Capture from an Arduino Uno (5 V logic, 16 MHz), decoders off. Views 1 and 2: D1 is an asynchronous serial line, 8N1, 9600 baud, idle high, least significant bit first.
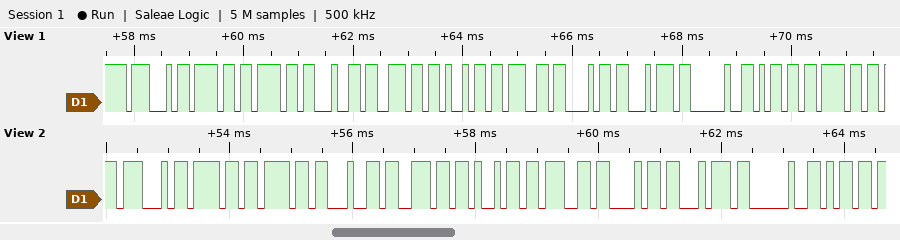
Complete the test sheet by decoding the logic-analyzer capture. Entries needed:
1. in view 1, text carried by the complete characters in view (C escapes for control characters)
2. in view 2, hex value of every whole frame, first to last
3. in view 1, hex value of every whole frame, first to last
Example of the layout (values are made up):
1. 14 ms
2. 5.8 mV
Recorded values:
1. "Goodnight mo"
2. 47 6F 6F 64 6E 69 67 68 74 20 6D
3. 47 6F 6F 64 6E 69 67 68 74 20 6D 6F
